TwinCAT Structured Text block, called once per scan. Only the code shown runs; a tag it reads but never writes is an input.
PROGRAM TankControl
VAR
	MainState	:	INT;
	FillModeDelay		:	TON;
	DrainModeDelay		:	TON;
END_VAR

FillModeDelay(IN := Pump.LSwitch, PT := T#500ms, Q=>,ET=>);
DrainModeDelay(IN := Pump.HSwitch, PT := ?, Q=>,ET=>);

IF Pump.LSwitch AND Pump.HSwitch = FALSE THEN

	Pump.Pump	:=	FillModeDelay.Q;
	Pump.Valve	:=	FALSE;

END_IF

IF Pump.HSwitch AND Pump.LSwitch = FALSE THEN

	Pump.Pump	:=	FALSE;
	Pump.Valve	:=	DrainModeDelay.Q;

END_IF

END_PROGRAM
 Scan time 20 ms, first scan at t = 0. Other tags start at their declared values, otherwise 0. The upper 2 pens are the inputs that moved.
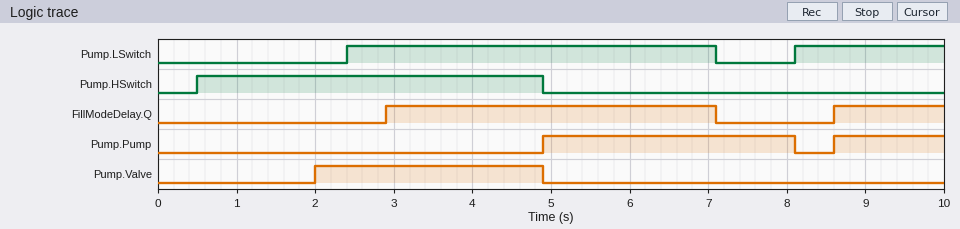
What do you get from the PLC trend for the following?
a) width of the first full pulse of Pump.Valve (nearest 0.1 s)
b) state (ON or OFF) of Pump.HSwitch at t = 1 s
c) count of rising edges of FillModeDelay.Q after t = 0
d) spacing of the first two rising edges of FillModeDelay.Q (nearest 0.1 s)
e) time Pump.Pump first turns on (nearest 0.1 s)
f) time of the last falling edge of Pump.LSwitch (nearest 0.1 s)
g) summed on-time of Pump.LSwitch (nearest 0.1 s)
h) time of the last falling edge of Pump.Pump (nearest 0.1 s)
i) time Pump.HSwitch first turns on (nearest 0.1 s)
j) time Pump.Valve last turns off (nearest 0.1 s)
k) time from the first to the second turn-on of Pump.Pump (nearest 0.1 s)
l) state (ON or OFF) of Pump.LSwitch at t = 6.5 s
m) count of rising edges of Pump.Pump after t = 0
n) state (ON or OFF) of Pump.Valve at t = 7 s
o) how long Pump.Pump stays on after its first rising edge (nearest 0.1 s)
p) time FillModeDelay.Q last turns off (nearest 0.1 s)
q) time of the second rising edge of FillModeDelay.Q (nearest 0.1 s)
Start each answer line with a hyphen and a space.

- 2.9 s
- ON
- 2
- 5.7 s
- 4.9 s
- 7.1 s
- 6.6 s
- 8.1 s
- 0.5 s
- 4.9 s
- 3.7 s
- ON
- 2
- OFF
- 3.2 s
- 7.1 s
- 8.6 s
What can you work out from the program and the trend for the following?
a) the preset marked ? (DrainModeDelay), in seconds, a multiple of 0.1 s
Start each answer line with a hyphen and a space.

- 1.5 s
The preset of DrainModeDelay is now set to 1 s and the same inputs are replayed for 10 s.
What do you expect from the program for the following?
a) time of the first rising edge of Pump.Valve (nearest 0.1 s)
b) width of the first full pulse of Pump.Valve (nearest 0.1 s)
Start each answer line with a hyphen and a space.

- 1.5 s
- 3.4 s
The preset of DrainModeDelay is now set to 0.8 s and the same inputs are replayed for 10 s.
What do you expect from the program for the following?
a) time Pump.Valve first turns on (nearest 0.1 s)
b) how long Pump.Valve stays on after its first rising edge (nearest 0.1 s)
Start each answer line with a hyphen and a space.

- 1.3 s
- 3.6 s
